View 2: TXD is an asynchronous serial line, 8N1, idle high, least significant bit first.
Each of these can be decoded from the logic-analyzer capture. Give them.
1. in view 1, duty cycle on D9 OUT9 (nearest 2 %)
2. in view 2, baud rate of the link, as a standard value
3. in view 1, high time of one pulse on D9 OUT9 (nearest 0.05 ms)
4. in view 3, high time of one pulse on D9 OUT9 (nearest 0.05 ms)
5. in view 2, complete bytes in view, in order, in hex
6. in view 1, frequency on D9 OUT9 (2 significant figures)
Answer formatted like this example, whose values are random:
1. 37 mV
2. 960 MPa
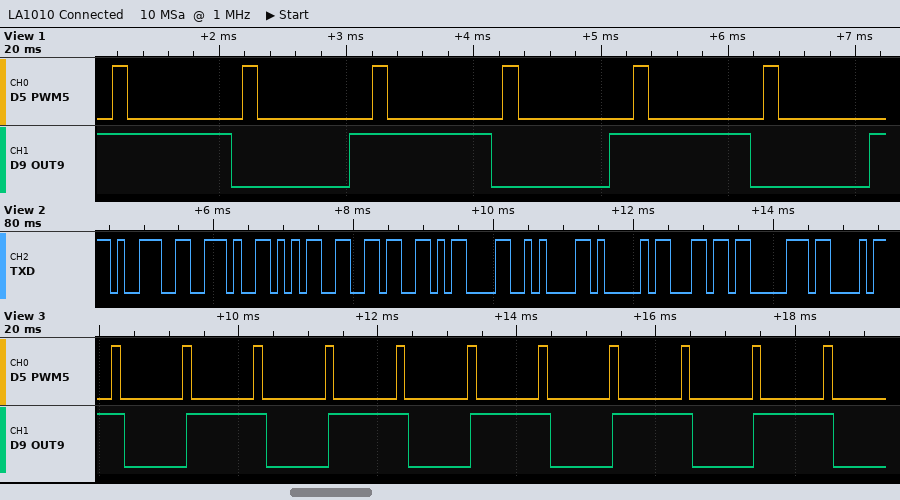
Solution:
1. 54 %
2. 9600 baud
3. 1.10 ms
4. 1.15 ms
5. 39 2E 35 36 0D 0A 41 6C 70
6. 490 Hz
